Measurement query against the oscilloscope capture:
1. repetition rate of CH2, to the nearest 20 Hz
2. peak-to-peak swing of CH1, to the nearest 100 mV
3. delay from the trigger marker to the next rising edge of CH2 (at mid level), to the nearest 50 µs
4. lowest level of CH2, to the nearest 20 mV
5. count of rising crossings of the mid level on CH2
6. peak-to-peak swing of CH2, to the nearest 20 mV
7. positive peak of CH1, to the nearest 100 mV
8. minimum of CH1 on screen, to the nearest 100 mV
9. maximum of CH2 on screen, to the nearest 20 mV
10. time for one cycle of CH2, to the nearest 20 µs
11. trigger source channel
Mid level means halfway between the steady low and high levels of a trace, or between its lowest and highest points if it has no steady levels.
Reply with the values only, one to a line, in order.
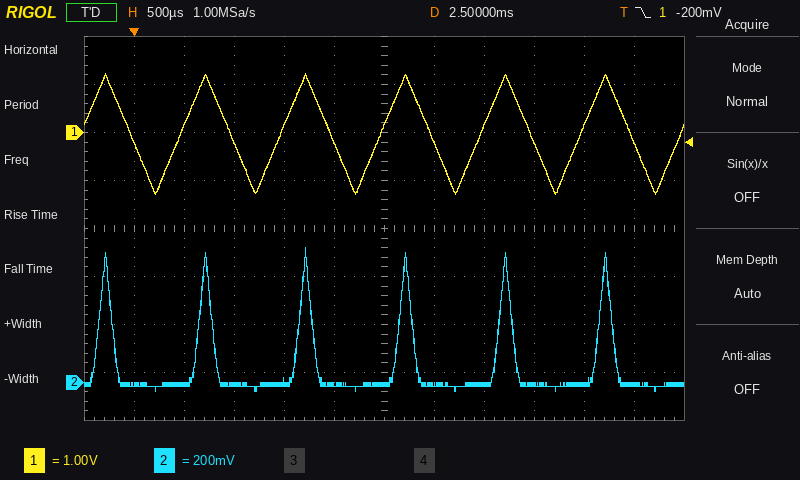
1.00 kHz
2.5 V
650 µs
-40 mV
6
600 mV
1.2 V
-1.3 V
560 mV
1.00 ms
CH1
